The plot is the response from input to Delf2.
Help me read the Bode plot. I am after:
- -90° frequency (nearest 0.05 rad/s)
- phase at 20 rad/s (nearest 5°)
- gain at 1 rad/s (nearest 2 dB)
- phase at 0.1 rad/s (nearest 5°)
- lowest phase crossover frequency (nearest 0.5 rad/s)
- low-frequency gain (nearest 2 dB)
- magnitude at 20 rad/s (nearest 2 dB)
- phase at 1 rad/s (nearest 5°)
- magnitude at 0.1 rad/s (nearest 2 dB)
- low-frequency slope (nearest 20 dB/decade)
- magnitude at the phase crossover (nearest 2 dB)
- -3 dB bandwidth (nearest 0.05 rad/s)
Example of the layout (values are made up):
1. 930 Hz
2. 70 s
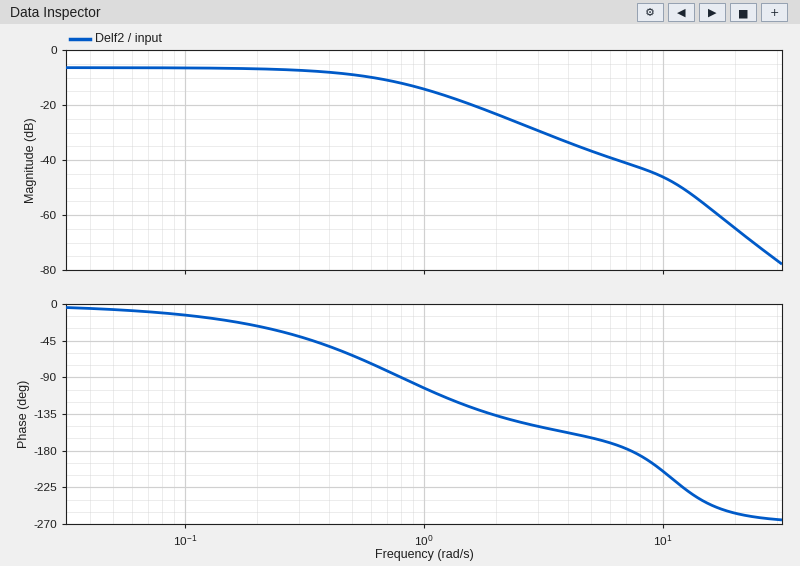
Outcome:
1. 0.80 rad/s
2. -255°
3. -14 dB
4. -15°
5. 7.5 rad/s
6. -6 dB
7. -64 dB
8. -105°
9. -6 dB
10. 0 dB/decade
11. -42 dB
12. 0.55 rad/s
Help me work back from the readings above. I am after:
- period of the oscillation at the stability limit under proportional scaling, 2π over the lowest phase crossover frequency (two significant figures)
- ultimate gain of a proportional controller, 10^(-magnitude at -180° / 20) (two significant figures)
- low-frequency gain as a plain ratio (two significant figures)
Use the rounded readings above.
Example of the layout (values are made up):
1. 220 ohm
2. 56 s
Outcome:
1. 0.84 s
2. 130
3. 0.50
